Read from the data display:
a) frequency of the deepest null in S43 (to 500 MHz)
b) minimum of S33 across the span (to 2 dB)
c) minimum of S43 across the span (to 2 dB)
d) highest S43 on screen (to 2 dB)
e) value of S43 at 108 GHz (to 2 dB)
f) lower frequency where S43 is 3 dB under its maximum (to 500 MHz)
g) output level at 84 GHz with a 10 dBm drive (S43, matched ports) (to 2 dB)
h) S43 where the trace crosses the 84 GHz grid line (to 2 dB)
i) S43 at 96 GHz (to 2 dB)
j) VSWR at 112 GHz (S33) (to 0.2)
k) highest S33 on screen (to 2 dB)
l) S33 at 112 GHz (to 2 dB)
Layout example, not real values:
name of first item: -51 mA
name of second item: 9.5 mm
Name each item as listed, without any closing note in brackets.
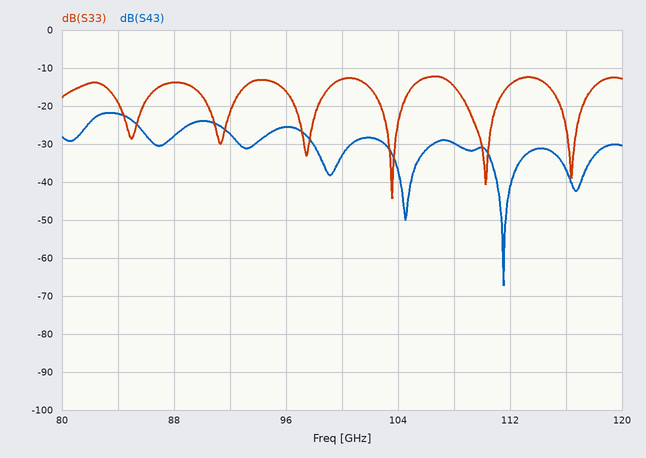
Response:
frequency of the deepest null in S43: 111.5 GHz
minimum of S33 across the span: -44 dB
minimum of S43 across the span: -68 dB
highest S43 on screen: -22 dB
value of S43 at 108 GHz: -30 dB
lower frequency where S43 is 3 dB under its maximum: 82.0 GHz
output level at 84 GHz with a 10 dBm drive (S43, matched ports): -12 dBm
S43 where the trace crosses the 84 GHz grid line: -22 dB
S43 at 96 GHz: -26 dB
VSWR at 112 GHz (S33): 1.4
highest S33 on screen: -12 dB
S33 at 112 GHz: -14 dB
